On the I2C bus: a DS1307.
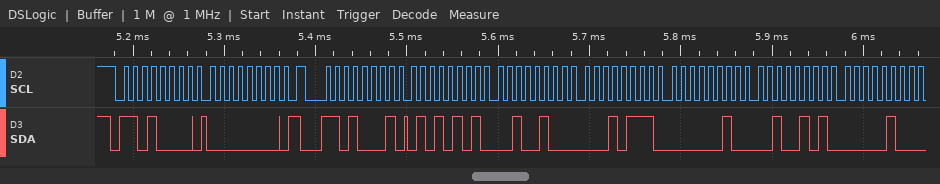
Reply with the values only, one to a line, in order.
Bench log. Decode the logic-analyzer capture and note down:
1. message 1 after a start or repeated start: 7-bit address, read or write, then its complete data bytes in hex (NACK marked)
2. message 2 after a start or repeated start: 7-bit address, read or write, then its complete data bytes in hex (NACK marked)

0x68 write: 00
0x68 read: 55 24 17 02 25 04
